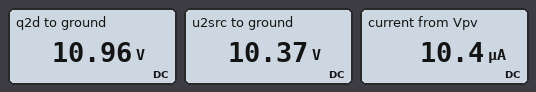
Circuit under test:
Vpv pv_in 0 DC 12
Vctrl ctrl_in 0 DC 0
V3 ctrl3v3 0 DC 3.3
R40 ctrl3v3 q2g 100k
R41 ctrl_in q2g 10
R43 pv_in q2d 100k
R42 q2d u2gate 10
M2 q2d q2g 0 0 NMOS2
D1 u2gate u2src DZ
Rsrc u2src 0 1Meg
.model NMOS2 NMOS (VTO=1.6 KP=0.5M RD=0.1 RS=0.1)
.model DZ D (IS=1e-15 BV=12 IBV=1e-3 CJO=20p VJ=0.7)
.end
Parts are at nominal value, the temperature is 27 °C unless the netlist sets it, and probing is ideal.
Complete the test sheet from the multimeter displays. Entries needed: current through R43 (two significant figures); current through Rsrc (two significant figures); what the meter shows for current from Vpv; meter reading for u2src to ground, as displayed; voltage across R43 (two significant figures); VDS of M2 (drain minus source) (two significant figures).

10 µA
10 µA
10.4 µA
10.37 V
1.0 V
11 V
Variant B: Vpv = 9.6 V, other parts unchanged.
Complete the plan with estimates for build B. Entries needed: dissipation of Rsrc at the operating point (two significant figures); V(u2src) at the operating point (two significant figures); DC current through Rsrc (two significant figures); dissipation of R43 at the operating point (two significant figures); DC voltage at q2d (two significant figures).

67 µW
8.2 V
8.2 µA
6.7 µW
8.8 V
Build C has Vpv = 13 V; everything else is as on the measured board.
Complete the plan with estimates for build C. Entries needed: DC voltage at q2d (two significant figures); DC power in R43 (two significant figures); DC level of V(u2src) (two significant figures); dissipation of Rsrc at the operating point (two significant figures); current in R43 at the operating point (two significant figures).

12 V
13 µW
11 V
130 µW
11 µA
